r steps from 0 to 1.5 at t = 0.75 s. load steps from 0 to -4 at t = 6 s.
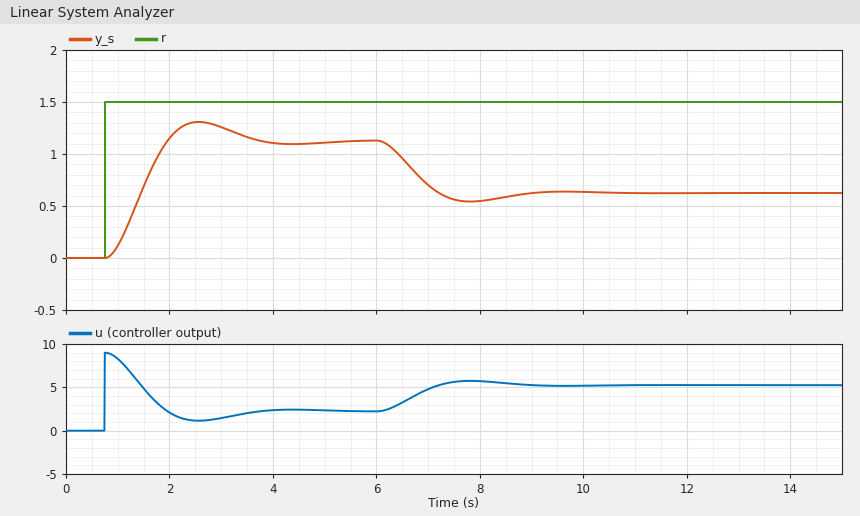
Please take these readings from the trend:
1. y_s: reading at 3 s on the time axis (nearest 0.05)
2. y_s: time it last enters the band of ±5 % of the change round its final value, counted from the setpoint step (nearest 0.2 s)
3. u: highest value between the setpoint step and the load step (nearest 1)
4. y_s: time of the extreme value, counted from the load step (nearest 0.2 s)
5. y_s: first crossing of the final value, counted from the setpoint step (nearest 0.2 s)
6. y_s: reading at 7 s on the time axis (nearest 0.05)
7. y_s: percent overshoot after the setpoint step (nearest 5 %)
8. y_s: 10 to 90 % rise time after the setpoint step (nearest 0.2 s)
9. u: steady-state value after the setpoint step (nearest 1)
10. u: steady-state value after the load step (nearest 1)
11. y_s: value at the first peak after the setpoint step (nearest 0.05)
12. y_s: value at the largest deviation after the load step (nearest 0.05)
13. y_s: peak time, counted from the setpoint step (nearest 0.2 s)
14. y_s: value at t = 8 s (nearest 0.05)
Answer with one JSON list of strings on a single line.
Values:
["1.25", "2.6 s", "9", "1.8 s", "1.2 s", "0.70", "15 %", "0.8 s", "2", "5", "1.30", "0.55", "1.8 s", "0.55"]
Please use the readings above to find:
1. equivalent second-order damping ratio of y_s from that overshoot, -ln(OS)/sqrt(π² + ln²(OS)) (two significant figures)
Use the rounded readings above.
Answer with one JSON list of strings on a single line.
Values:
["0.52"]
